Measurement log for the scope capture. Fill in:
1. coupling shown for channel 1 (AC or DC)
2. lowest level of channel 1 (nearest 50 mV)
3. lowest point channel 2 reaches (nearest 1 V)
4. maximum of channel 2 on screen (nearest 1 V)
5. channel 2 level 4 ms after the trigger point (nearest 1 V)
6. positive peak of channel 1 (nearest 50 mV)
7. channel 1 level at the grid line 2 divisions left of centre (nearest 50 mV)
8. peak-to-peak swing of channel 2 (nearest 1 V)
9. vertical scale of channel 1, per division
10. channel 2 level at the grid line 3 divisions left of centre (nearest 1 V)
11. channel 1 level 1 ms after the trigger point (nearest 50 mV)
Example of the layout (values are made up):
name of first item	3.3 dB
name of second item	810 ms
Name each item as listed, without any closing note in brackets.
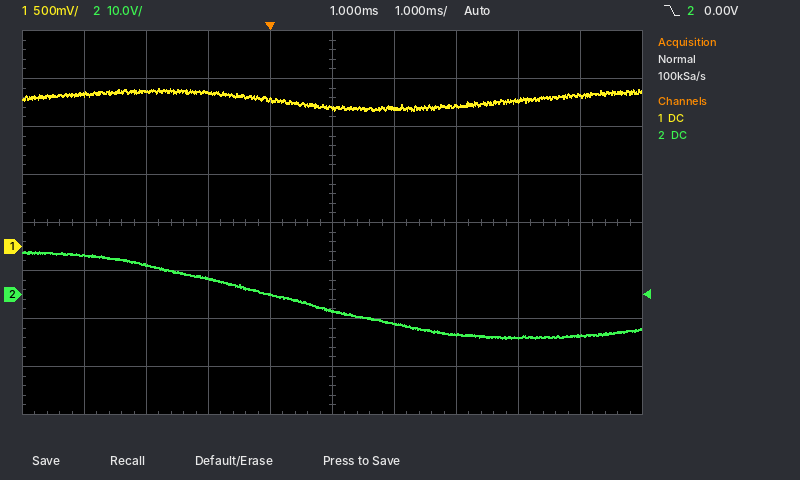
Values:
coupling shown for channel 1	DC
lowest level of channel 1	1.40 V
lowest point channel 2 reaches	-9 V
maximum of channel 2 on screen	9 V
channel 2 level 4 ms after the trigger point	-9 V
positive peak of channel 1	1.65 V
channel 1 level at the grid line 2 divisions left of centre	1.60 V
peak-to-peak swing of channel 2	18 V
vertical scale of channel 1, per division	500 mV
channel 2 level at the grid line 3 divisions left of centre	6 V
channel 1 level 1 ms after the trigger point	1.45 V
